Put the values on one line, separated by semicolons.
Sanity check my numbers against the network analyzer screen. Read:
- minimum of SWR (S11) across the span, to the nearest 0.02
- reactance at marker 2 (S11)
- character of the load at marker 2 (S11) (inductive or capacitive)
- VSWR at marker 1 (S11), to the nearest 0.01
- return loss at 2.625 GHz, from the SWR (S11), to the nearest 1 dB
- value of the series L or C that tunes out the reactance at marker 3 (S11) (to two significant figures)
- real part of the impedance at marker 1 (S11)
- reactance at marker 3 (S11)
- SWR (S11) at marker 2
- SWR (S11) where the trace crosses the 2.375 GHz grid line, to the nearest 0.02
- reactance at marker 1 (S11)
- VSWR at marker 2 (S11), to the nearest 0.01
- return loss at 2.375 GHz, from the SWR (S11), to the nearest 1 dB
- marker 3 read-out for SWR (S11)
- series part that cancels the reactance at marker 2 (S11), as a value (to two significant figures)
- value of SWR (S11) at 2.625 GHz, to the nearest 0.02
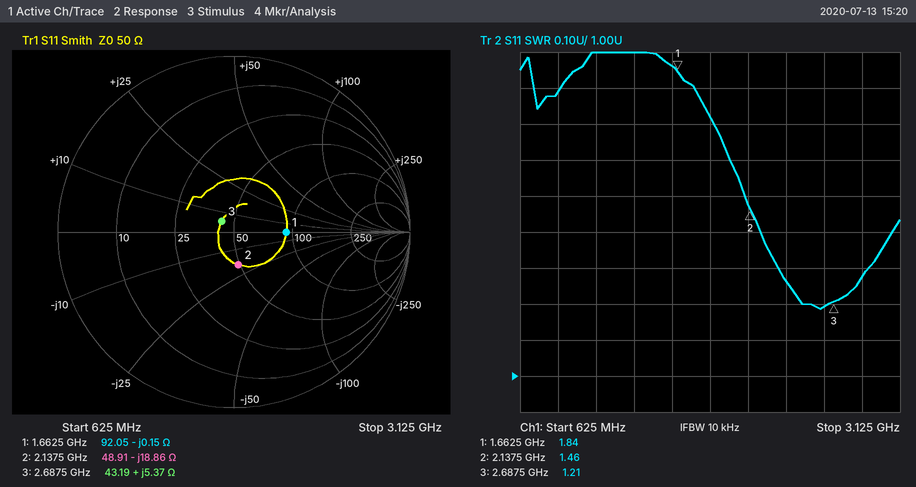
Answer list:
1.18; -18.86 Ω; capacitive; 1.84; 21 dB; 11 pF; 92.05 Ω; +5.37 Ω; 1.46; 1.26; -0.15 Ω; 1.46; 19 dB; 1.21; 1.4 nH; 1.20
